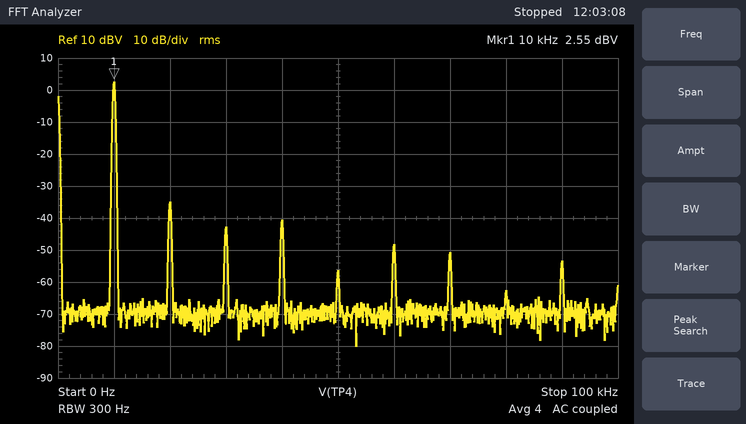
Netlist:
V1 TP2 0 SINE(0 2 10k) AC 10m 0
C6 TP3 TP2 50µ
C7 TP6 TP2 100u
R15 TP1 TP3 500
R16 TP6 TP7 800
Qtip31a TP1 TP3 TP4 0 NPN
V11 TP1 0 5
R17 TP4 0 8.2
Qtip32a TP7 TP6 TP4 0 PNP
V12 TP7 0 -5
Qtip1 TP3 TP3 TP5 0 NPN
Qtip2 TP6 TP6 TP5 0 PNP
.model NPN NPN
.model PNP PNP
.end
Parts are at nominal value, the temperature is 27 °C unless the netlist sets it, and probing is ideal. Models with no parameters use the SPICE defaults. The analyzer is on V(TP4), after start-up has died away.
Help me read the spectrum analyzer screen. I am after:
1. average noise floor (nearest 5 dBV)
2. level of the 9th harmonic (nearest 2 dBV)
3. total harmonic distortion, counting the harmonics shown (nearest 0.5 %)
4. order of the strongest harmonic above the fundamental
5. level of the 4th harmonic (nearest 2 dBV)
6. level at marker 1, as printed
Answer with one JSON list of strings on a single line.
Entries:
["-70 dBV", "-54 dBV", "1.5 %", "2", "-40 dBV", "2.55 dBV"]
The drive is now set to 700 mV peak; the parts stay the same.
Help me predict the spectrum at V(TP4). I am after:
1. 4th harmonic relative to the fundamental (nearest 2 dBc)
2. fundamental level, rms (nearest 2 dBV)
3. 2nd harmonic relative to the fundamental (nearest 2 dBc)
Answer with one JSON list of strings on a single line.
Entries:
["-54 dBc", "-6 dBV", "-36 dBc"]
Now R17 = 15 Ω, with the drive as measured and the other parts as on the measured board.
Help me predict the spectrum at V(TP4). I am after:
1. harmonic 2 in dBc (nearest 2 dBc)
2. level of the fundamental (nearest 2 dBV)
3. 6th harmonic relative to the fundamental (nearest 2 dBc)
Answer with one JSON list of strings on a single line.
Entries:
["-40 dBc", "2 dBV", "-58 dBc"]
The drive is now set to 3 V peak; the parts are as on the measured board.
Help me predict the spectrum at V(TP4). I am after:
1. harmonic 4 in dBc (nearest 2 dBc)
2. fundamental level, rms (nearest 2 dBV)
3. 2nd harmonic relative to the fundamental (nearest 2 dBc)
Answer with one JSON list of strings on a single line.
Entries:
["-46 dBc", "6 dBV", "-42 dBc"]
